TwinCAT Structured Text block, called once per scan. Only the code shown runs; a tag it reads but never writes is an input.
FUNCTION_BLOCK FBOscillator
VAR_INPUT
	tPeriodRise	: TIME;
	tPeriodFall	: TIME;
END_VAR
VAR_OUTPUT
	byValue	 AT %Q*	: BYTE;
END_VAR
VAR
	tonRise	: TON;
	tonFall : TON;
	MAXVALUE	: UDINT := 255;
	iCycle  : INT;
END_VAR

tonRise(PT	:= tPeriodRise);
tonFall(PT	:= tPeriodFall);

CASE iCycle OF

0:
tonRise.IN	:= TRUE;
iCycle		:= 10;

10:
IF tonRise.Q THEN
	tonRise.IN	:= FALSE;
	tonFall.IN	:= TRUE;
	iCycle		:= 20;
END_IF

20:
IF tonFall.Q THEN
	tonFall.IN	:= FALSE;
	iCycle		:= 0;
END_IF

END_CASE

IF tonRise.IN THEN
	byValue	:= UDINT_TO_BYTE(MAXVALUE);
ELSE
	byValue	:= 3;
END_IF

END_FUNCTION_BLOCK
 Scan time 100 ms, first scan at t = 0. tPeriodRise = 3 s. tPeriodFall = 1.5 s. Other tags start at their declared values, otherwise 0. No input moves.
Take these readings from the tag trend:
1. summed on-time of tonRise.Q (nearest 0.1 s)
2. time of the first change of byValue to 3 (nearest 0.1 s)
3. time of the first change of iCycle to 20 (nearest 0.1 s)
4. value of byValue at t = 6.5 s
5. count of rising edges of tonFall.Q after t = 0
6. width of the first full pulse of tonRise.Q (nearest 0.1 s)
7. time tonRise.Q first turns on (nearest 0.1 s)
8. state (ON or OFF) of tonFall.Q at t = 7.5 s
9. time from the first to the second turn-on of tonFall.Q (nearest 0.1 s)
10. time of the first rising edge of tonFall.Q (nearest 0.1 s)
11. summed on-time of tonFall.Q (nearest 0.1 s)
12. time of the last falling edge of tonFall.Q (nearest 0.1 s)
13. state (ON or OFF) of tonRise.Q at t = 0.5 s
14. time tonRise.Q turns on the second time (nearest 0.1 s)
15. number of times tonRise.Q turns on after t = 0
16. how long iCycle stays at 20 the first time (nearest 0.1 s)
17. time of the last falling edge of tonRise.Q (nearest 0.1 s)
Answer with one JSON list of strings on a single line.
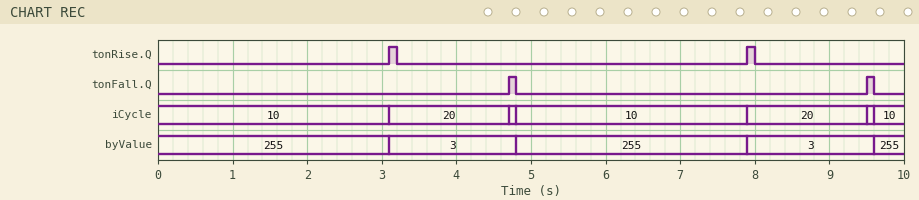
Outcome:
["0.2 s", "3.1 s", "3.1 s", "255", "2", "0.1 s", "3.1 s", "OFF", "4.8 s", "4.7 s", "0.2 s", "9.6 s", "OFF", "7.9 s", "2", "1.6 s", "8.0 s"]
